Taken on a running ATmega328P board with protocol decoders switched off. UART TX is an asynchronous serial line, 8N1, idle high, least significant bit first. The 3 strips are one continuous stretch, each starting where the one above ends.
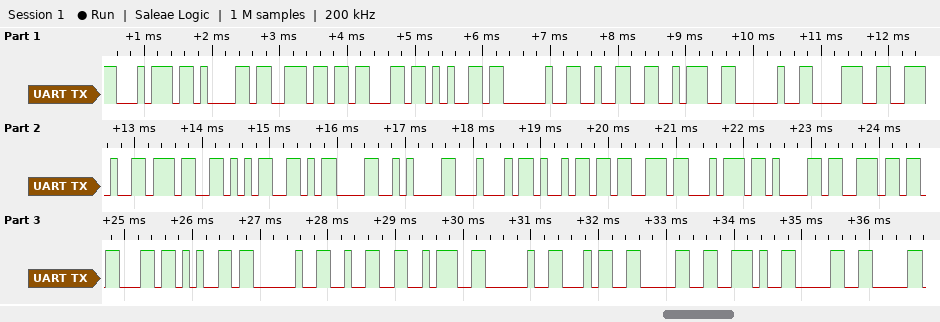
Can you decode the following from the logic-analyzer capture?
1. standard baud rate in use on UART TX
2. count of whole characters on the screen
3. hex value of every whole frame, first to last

9600 baud
31
74 61 6E 63 65 20 32 3A 20 38 2E 37 35 0D 0A 44 69 73 74 61 6E 63 65 20 32 3A 20 34 30 2E 30
